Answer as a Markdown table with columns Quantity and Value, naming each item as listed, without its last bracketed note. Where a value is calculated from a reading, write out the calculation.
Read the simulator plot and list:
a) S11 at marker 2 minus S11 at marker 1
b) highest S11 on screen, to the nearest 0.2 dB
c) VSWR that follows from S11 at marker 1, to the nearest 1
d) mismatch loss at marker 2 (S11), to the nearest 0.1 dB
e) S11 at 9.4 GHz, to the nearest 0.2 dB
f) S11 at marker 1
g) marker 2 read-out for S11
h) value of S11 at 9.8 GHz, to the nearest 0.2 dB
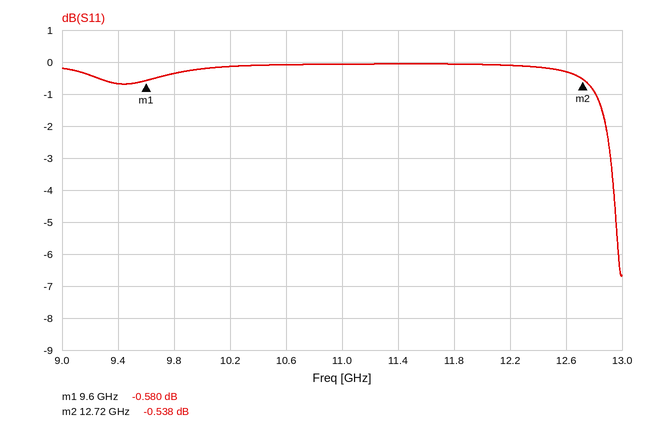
| Quantity | Value |
|---|---|
| S11 at marker 2 minus S11 at marker 1 | -0.538 − (-0.58) = 0.042 dB |
| highest S11 on screen, to the nearest 0.2 dB | 0.0 dB |
| VSWR that follows from S11 at marker 1, to the nearest 1 | (1 + 0.9354)/(1 − 0.9354) ≈ 30 |
| mismatch loss at marker 2 (S11), to the nearest 0.1 dB | −10 log10(1 − 10^(-0.538/10)) ≈ 9.3 dB |
| S11 at 9.4 GHz, to the nearest 0.2 dB | -0.6 dB |
| S11 at marker 1 | -0.580 dB |
| marker 2 read-out for S11 | -0.538 dB |
| value of S11 at 9.8 GHz, to the nearest 0.2 dB | -0.4 dB |
